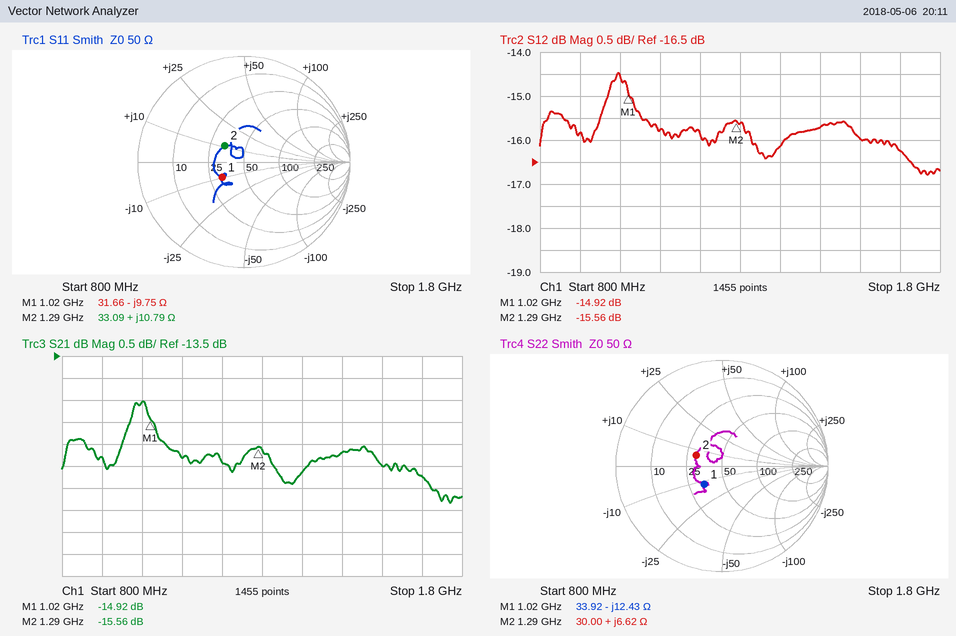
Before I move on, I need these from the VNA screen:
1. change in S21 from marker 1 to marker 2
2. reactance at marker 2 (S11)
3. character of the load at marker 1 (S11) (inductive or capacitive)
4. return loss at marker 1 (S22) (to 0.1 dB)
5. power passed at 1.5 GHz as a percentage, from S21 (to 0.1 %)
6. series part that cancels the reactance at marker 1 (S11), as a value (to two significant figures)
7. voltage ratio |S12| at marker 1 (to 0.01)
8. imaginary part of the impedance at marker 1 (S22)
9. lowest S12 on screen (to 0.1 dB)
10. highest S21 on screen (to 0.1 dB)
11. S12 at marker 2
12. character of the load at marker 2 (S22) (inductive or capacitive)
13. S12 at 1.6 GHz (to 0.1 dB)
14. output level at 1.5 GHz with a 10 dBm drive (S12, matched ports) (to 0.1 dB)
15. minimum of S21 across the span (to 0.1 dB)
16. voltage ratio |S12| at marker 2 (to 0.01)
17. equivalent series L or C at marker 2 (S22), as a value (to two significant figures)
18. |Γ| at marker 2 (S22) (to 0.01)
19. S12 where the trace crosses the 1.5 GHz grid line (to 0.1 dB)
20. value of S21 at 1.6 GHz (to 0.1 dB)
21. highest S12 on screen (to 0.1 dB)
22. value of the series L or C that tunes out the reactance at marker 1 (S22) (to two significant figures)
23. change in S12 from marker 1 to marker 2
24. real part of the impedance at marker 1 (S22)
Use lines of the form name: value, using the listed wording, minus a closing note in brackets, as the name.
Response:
change in S21 from marker 1 to marker 2: -0.64 dB
reactance at marker 2: +10.79 Ω
character of the load at marker 1 (S11): capacitive
return loss at marker 1 (S22): 12.4 dB
power passed at 1.5 GHz as a percentage, from S21: 2.7 %
series part that cancels the reactance at marker 1 (S11), as a value: 1.5 nH
voltage ratio |S12| at marker 1: 0.18
imaginary part of the impedance at marker 1: -12.43 Ω
lowest S12 on screen: -16.8 dB
highest S21 on screen: -14.5 dB
S12 at marker 2: -15.56 dB
character of the load at marker 2 (S22): inductive
S12 at 1.6 GHz: -16.0 dB
output level at 1.5 GHz with a 10 dBm drive (S12, matched ports): -5.7 dBm
minimum of S21 across the span: -16.8 dB
voltage ratio |S12| at marker 2: 0.17
equivalent series L or C at marker 2 (S22), as a value: 820 pH
|Γ| at marker 2 (S22): 0.26
S12 where the trace crosses the 1.5 GHz grid line: -15.7 dB
value of S21 at 1.6 GHz: -16.0 dB
highest S12 on screen: -14.5 dB
value of the series L or C that tunes out the reactance at marker 1 (S22): 1.9 nH
change in S12 from marker 1 to marker 2: -0.64 dB
real part of the impedance at marker 1: 33.92 Ω
